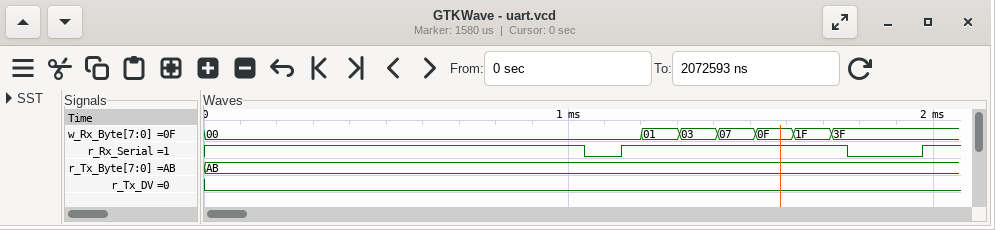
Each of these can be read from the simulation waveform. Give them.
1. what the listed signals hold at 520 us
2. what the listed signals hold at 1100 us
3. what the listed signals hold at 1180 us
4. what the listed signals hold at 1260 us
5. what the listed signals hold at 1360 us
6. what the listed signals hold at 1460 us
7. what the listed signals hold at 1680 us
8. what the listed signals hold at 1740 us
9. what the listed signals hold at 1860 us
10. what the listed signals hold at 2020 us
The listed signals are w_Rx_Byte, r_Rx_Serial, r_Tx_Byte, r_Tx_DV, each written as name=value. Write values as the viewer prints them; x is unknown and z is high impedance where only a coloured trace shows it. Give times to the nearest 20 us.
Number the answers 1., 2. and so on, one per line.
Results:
1. w_Rx_Byte=00, r_Rx_Serial=1, r_Tx_Byte=AB, r_Tx_DV=0
2. w_Rx_Byte=00, r_Rx_Serial=0, r_Tx_Byte=AB, r_Tx_DV=0
3. w_Rx_Byte=00, r_Rx_Serial=1, r_Tx_Byte=AB, r_Tx_DV=0
4. w_Rx_Byte=01, r_Rx_Serial=1, r_Tx_Byte=AB, r_Tx_DV=0
5. w_Rx_Byte=03, r_Rx_Serial=1, r_Tx_Byte=AB, r_Tx_DV=0
6. w_Rx_Byte=07, r_Rx_Serial=1, r_Tx_Byte=AB, r_Tx_DV=0
7. w_Rx_Byte=1F, r_Rx_Serial=1, r_Tx_Byte=AB, r_Tx_DV=0
8. w_Rx_Byte=3F, r_Rx_Serial=1, r_Tx_Byte=AB, r_Tx_DV=0
9. w_Rx_Byte=3F, r_Rx_Serial=0, r_Tx_Byte=AB, r_Tx_DV=0
10. w_Rx_Byte=3F, r_Rx_Serial=1, r_Tx_Byte=AB, r_Tx_DV=0
